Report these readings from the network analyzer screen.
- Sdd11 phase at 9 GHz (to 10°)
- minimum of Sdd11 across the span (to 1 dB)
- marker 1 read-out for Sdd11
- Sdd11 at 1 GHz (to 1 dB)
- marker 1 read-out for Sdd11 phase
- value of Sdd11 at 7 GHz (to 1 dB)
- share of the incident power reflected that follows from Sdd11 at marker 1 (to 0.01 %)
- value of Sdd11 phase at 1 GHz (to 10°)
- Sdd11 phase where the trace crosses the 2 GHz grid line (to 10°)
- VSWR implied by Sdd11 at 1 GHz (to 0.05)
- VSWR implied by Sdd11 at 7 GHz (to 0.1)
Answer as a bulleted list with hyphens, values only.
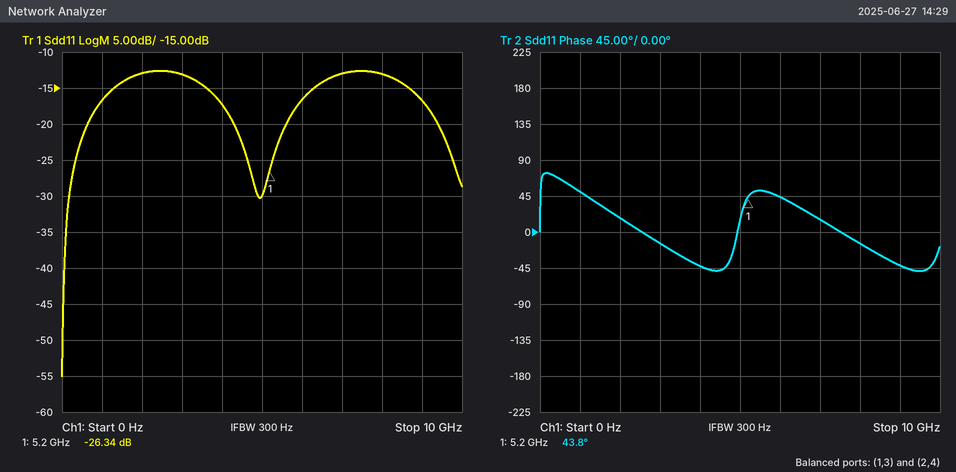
- -40°
- -55 dB
- -26.34 dB
- -17 dB
- 43.8°
- -13 dB
- 0.23 %
- 50°
- 20°
- 1.35
- 1.6
